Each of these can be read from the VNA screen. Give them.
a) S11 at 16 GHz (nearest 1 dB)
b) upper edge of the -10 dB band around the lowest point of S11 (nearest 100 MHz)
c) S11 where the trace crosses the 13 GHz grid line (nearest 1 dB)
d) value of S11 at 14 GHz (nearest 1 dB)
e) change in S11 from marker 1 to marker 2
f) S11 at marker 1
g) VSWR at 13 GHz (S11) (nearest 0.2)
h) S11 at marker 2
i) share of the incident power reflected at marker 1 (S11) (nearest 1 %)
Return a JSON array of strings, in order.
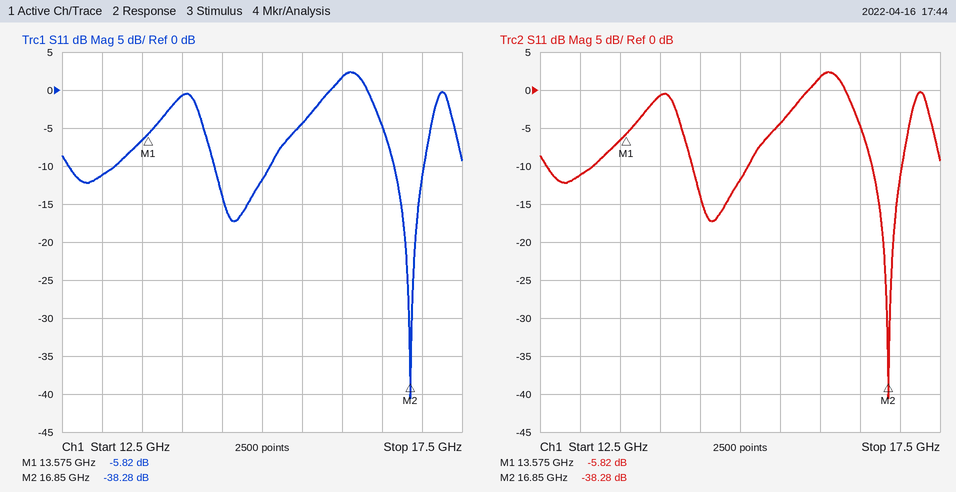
["2 dB", "17.0 GHz", "-11 dB", "-1 dB", "-32.46 dB", "-5.82 dB", "1.8", "-38.28 dB", "26 %"]
